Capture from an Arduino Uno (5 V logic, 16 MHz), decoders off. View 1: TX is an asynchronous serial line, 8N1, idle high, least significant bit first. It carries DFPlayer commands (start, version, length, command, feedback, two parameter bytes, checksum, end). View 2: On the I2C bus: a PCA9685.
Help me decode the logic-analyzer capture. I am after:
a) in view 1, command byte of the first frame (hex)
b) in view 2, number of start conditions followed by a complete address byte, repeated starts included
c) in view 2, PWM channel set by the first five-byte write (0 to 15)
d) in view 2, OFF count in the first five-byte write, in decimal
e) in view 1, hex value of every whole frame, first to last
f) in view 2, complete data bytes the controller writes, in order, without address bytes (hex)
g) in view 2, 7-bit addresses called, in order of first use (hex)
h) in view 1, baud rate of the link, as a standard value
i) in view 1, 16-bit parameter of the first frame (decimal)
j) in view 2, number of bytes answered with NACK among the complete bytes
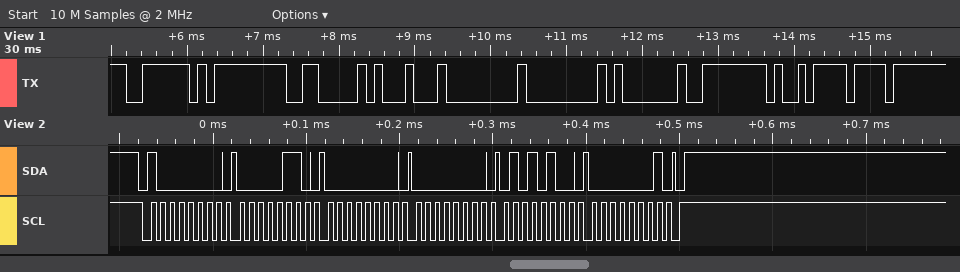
0x11
1
0
340
7E FF 06 11 00 00 01 FE E9 EF
06 00 00 54 01
0x40
9600 baud
1
0
